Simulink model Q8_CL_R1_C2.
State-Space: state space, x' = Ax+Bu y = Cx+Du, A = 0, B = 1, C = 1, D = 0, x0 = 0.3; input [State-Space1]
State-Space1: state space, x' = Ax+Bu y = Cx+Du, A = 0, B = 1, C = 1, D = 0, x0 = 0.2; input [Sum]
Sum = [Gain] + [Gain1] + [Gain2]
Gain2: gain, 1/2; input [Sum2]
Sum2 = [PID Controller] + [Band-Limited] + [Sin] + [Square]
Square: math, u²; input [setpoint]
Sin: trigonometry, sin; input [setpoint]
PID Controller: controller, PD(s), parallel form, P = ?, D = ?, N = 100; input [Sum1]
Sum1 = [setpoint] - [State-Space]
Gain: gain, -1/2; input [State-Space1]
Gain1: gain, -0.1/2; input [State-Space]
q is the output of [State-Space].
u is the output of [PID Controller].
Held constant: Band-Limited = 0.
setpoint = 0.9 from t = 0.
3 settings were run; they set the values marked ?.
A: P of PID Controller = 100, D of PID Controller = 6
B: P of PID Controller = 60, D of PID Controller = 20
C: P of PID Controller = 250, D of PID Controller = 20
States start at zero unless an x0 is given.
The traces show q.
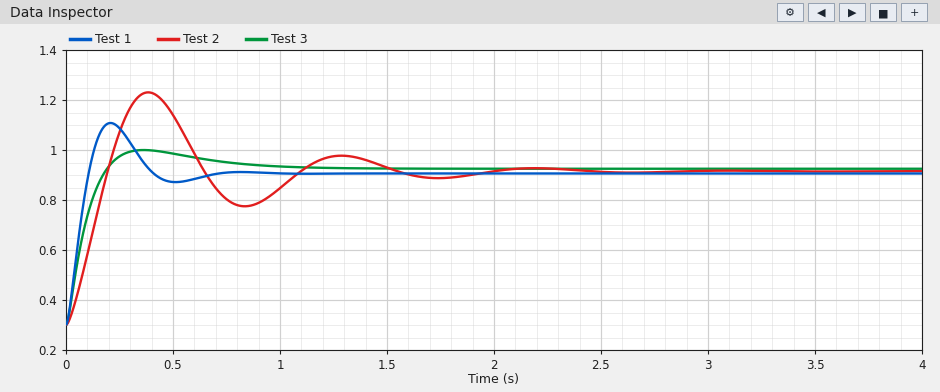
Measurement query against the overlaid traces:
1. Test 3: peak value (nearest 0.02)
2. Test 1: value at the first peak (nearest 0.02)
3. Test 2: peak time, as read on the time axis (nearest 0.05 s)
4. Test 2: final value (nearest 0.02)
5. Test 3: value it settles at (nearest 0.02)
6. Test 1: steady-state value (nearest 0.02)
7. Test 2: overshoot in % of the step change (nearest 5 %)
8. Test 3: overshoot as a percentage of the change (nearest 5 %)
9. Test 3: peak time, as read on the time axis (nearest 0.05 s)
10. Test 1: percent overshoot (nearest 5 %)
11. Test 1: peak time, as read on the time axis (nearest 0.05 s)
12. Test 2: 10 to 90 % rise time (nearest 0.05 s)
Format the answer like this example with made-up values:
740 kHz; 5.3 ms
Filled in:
1.00; 1.10; 0.40 s; 0.92; 0.92; 0.90; 50 %; 10 %; 0.35 s; 35 %; 0.20 s; 0.15 s
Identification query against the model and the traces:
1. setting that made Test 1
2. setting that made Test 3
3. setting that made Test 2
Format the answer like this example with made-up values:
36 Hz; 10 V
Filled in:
C; B; A
